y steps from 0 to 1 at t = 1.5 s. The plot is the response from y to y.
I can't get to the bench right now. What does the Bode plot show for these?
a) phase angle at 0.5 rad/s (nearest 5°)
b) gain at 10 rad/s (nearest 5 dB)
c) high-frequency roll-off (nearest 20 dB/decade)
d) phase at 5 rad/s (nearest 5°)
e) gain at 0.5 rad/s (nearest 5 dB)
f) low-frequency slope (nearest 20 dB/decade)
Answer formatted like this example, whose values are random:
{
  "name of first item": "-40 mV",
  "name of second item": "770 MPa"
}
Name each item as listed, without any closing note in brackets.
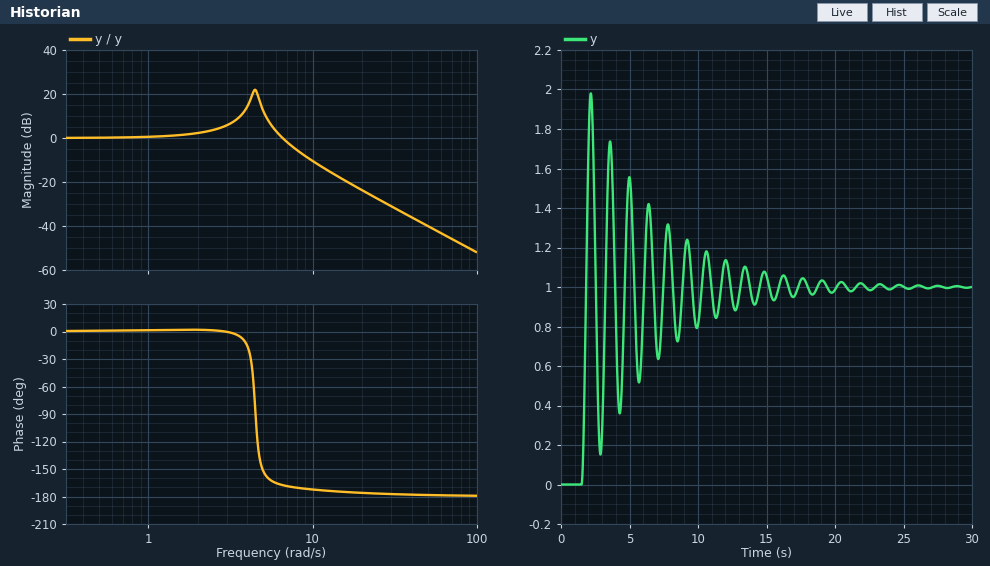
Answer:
{
  "phase angle at 0.5 rad/s": "0°",
  "gain at 10 rad/s": "-10 dB",
  "high-frequency roll-off": "-40 dB/decade",
  "phase at 5 rad/s": "-150°",
  "gain at 0.5 rad/s": "0 dB",
  "low-frequency slope": "0 dB/decade"
}
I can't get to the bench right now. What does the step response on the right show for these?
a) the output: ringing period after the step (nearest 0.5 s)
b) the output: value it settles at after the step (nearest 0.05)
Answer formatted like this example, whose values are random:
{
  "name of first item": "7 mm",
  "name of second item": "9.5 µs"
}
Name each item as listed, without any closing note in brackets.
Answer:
{
  "the output: ringing period after the step": "1.5 s",
  "the output: value it settles at after the step": "1.00"
}
